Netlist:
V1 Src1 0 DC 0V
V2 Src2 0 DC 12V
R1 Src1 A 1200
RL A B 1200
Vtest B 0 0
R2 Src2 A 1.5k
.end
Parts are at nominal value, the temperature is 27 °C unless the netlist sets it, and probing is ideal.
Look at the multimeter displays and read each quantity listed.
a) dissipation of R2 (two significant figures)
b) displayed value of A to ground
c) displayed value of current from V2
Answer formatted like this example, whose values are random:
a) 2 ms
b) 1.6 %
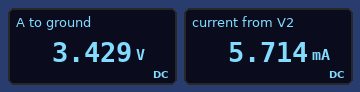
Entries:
a) 49 mW
b) 3.429 V
c) 5.714 mA
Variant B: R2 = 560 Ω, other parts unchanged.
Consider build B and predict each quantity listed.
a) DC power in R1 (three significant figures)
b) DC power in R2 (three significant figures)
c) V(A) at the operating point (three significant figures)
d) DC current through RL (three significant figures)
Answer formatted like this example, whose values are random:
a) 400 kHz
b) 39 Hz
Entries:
a) 32.1 mW
b) 59.9 mW
c) 6.21 V
d) 5.17 mA
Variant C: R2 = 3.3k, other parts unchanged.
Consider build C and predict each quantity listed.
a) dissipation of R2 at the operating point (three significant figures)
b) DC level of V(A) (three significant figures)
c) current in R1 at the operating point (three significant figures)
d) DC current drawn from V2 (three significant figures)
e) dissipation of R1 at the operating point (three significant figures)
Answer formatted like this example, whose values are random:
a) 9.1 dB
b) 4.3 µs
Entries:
a) 31.2 mW
b) 1.85 V
c) 1.54 mA
d) 3.08 mA
e) 2.84 mW
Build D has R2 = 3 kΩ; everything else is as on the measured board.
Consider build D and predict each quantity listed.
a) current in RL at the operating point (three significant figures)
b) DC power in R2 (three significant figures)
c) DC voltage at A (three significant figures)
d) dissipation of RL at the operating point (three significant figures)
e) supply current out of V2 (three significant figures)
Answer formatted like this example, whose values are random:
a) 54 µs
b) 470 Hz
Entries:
a) 1.67 mA
b) 33.3 mW
c) 2.00 V
d) 3.33 mW
e) 3.33 mA
